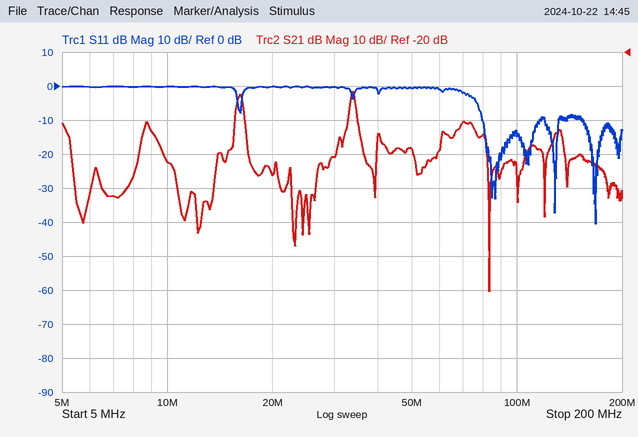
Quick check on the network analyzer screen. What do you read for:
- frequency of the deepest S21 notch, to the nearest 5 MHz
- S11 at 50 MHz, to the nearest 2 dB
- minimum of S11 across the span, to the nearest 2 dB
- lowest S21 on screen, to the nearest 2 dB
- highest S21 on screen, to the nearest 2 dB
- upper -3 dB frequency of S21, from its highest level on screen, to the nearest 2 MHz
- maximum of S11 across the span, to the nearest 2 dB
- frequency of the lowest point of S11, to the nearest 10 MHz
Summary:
85 MHz
0 dB
-40 dB
-90 dB
-32 dB
34 MHz
0 dB
170 MHz
